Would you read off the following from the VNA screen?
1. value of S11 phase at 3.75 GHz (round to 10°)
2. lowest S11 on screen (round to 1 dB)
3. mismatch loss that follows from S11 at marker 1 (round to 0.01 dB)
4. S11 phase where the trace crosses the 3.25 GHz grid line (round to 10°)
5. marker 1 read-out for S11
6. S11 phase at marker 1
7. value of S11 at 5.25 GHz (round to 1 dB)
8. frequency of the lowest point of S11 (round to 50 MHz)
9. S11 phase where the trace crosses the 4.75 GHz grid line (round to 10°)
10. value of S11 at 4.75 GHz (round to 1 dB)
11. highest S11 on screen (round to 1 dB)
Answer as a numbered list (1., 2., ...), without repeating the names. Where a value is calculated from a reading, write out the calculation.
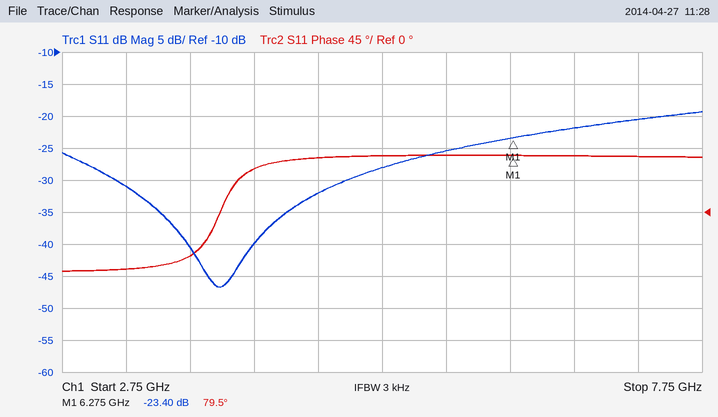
1. -60°
2. -47 dB
3. −10 log10(1 − 10^(-23.4/10)) ≈ 0.02 dB
4. -80°
5. -23.40 dB
6. 79.5°
7. -28 dB
8. 4.00 GHz
9. 80°
10. -32 dB
11. -19 dB
